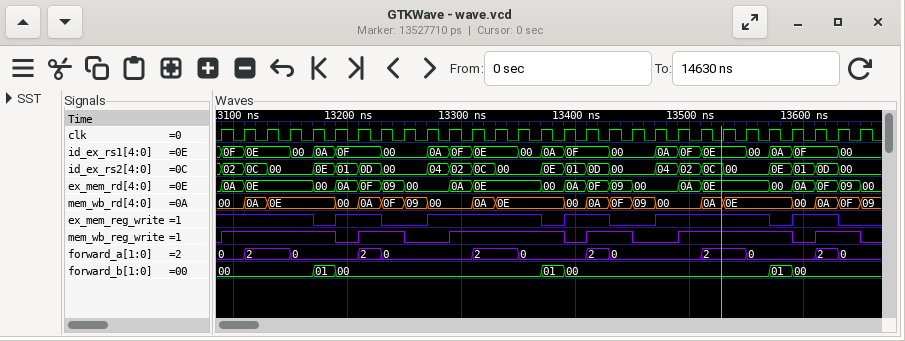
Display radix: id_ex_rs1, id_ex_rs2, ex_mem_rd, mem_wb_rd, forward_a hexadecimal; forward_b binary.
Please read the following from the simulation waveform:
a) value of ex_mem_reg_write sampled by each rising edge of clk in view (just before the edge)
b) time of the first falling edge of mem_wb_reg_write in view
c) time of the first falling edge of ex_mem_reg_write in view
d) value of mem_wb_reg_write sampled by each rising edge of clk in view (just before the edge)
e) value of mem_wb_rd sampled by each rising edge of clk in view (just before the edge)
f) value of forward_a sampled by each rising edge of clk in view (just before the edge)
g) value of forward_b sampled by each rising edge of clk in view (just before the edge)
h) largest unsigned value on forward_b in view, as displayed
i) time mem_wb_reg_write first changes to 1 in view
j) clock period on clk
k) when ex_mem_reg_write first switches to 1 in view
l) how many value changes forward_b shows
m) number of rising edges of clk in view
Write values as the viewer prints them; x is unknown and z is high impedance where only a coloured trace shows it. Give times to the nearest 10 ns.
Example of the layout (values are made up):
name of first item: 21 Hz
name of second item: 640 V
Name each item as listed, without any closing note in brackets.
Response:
value of ex_mem_reg_write sampled by each rising edge of clk in view: 1 1 1 1 1 0 1 1 0 0 1 1 1 1 1 0 1 1 0 0 1 1 1 1 1 0 1 1 0
time of the first falling edge of mem_wb_reg_write in view: 13190 ns
time of the first falling edge of ex_mem_reg_write in view: 13170 ns
value of mem_wb_reg_write sampled by each rising edge of clk in view: 0 1 1 1 1 1 0 1 1 0 0 1 1 1 1 1 0 1 1 0 0 1 1 1 1 1 0 1 1
value of mem_wb_rd sampled by each rising edge of clk in view: 00, 00, 0A, 0E, 0E, 0E, 00, 0A, 0F, 09, 00, 00, 0A, 0E, 0E, 0E, 00, 0A, 0F, 09, 00, 00, 0A, 0E, 0E, 0E, 00, 0A, 0F
value of forward_a sampled by each rising edge of clk in view: 0, 0, 2, 2, 0, 0, 0, 2, 0, 0, 0, 0, 2, 2, 0, 0, 0, 2, 0, 0, 0, 0, 2, 2, 0, 0, 0, 2, 0
value of forward_b sampled by each rising edge of clk in view: 00, 00, 00, 00, 00, 01, 00, 00, 00, 00, 00, 00, 00, 00, 00, 01, 00, 00, 00, 00, 00, 00, 00, 00, 00, 01, 00, 00, 00
largest unsigned value on forward_b in view, as displayed: 01
time mem_wb_reg_write first changes to 1 in view: 13090 ns
clock period on clk: 20 ns
when ex_mem_reg_write first switches to 1 in view: 13190 ns
how many value changes forward_b shows: 6
number of rising edges of clk in view: 29
